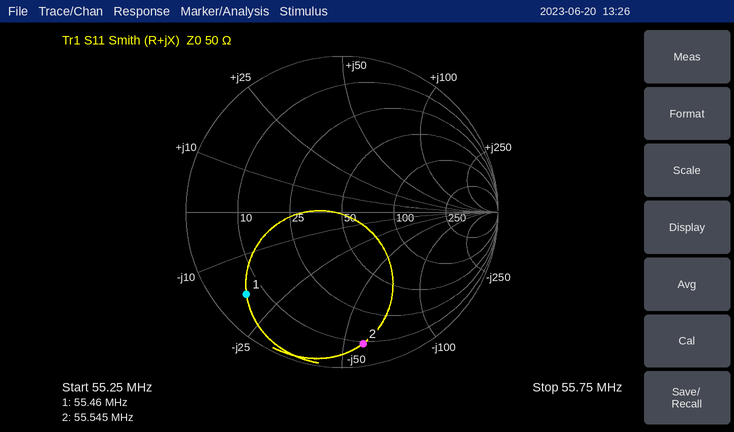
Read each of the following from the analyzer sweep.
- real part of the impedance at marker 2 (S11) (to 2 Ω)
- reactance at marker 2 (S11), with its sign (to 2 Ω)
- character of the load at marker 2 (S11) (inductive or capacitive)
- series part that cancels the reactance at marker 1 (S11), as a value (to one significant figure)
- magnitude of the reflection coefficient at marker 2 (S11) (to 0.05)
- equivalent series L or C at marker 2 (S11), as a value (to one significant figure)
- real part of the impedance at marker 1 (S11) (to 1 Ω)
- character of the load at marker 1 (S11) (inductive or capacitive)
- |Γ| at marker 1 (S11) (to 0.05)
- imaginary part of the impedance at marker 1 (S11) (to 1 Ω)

10 Ω
-58 Ω
capacitive
50 nH
0.85
50 pF
6 Ω
capacitive
0.80
-18 Ω
